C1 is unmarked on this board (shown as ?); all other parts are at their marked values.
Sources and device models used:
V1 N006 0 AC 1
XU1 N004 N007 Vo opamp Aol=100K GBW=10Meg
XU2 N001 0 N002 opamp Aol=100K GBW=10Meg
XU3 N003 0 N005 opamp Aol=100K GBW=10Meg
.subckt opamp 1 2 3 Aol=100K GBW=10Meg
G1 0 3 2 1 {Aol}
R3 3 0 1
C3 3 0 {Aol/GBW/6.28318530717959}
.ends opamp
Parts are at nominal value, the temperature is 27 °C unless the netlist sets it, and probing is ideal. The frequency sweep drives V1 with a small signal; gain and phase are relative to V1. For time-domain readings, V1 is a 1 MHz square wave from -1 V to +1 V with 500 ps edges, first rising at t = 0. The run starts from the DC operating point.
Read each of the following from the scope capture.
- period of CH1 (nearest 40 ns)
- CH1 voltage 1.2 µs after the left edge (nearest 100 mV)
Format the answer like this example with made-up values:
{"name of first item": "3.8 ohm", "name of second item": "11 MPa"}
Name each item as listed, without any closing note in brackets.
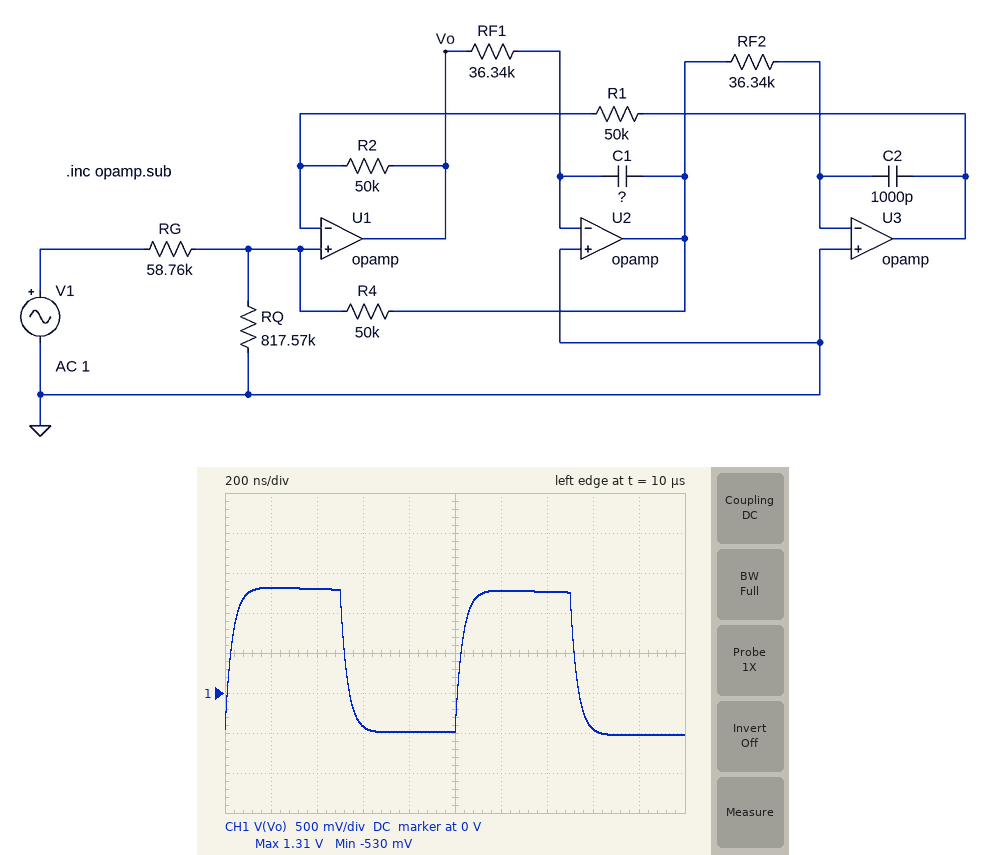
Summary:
{"period of CH1": "1.00 µs", "CH1 voltage 1.2 µs after the left edge": "1.3 V"}
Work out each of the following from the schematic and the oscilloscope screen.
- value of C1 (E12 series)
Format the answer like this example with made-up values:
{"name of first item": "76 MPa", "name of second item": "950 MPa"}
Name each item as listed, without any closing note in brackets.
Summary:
{"value of C1": "470 pF"}
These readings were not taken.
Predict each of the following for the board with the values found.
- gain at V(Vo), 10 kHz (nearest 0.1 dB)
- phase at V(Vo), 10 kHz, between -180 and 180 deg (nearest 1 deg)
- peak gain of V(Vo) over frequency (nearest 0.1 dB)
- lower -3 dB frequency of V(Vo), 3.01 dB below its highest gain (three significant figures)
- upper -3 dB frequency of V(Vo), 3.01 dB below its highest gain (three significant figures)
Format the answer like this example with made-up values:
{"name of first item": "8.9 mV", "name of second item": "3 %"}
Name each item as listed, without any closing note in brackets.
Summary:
{"gain at V(Vo), 10 kHz": "-2.1 dB", "phase at V(Vo), 10 kHz, between -180 and 180 deg": "59 deg", "peak gain of V(Vo) over frequency": "-1.0 dB", "lower -3 dB frequency of V(Vo), 3.01 dB below its highest gain": "6.93 kHz", "upper -3 dB frequency of V(Vo), 3.01 dB below its highest gain": "4.99 MHz"}
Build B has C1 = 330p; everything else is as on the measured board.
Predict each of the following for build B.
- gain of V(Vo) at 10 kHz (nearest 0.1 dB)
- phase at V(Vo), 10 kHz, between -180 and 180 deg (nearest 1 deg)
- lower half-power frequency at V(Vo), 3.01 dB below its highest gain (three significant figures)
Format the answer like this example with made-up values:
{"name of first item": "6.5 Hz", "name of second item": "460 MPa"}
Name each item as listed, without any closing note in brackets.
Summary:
{"gain of V(Vo) at 10 kHz": "-4.2 dB", "phase at V(Vo), 10 kHz, between -180 and 180 deg": "73 deg", "lower half-power frequency at V(Vo), 3.01 dB below its highest gain": "10.4 kHz"}
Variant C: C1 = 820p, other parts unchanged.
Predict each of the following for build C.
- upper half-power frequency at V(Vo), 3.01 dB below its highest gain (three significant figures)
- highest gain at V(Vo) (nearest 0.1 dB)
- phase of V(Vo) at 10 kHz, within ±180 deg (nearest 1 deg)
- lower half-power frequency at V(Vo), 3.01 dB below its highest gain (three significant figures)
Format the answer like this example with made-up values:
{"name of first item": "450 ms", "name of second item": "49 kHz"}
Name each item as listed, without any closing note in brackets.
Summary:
{"upper half-power frequency at V(Vo), 3.01 dB below its highest gain": "4.40 MHz", "highest gain at V(Vo)": "-0.5 dB", "phase of V(Vo) at 10 kHz, within ±180 deg": "36 deg", "lower half-power frequency at V(Vo), 3.01 dB below its highest gain": "4.28 kHz"}
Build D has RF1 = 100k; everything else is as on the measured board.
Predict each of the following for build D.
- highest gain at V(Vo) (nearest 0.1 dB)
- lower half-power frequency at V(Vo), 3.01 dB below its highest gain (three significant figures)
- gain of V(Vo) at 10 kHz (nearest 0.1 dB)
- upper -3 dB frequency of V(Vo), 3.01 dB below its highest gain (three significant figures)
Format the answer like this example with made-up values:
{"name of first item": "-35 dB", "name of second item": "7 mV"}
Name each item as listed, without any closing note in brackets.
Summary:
{"highest gain at V(Vo)": "0.8 dB", "lower half-power frequency at V(Vo), 3.01 dB below its highest gain": "3.26 kHz", "gain of V(Vo) at 10 kHz": "-0.3 dB", "upper -3 dB frequency of V(Vo), 3.01 dB below its highest gain": "2.88 MHz"}
